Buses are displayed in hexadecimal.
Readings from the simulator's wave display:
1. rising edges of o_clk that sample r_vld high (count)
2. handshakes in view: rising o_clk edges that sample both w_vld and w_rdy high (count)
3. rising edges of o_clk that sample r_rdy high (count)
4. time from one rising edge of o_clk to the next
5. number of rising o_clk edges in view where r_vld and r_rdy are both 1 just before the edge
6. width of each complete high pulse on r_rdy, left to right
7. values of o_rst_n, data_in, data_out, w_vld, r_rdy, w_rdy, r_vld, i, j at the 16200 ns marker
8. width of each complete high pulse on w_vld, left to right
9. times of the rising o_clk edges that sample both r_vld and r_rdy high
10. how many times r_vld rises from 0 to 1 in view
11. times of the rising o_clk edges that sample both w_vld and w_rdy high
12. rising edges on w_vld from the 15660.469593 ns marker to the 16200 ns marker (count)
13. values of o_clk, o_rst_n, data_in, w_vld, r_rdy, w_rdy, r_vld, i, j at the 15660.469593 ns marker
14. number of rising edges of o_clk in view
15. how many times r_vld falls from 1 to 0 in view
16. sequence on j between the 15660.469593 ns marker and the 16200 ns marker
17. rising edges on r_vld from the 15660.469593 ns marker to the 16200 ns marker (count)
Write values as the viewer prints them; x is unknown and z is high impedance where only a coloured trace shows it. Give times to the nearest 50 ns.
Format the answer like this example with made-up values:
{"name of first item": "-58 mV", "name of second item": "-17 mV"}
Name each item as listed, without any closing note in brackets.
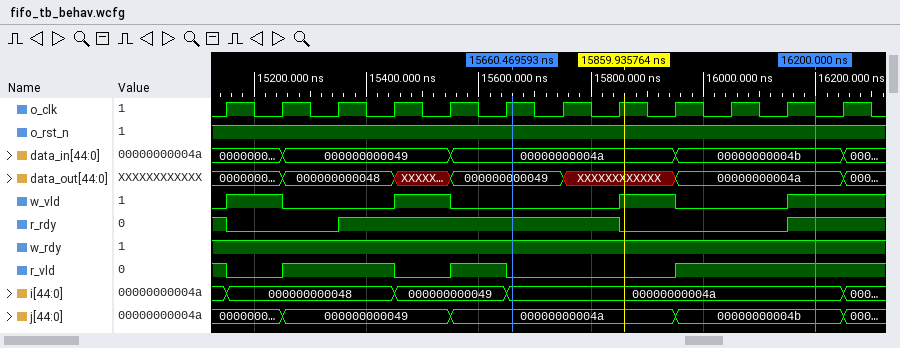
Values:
{"rising edges of o_clk that sample r_vld high": "7", "handshakes in view: rising o_clk edges that sample both w_vld and w_rdy high": "4", "rising edges of o_clk that sample r_rdy high": "7", "time from one rising edge of o_clk to the next": "100 ns", "number of rising o_clk edges in view where r_vld and r_rdy are both 1 just before the edge": "4", "width of each complete high pulse on r_rdy, left to right": "500 ns", "values of o_rst_n, data_in, data_out, w_vld, r_rdy, w_rdy, r_vld, i, j at the 16200 ns marker": "o_rst_n=1, data_in=00000000004b, data_out=00000000004a, w_vld=1, r_rdy=1, w_rdy=1, r_vld=1, i=00000000004a, j=00000000004b", "width of each complete high pulse on w_vld, left to right": "100 ns, 100 ns, 100 ns", "times of the rising o_clk edges that sample both r_vld and r_rdy high": "15150 ns, 15450 ns, 15650 ns, 16250 ns", "how many times r_vld rises from 0 to 1 in view": "3", "times of the rising o_clk edges that sample both w_vld and w_rdy high": "15250 ns, 15550 ns, 15950 ns, 16250 ns", "rising edges on w_vld from the 15660.469593 ns marker to the 16200 ns marker": "2", "values of o_clk, o_rst_n, data_in, w_vld, r_rdy, w_rdy, r_vld, i, j at the 15660.469593 ns marker": "o_clk=1, o_rst_n=1, data_in=00000000004a, w_vld=0, r_rdy=1, w_rdy=1, r_vld=0, i=00000000004a, j=00000000004a", "number of rising edges of o_clk in view": "12", "how many times r_vld falls from 1 to 0 in view": "3", "sequence on j between the 15660.469593 ns marker and the 16200 ns marker": "00000000004a, 00000000004b", "rising edges on r_vld from the 15660.469593 ns marker to the 16200 ns marker": "1"}
